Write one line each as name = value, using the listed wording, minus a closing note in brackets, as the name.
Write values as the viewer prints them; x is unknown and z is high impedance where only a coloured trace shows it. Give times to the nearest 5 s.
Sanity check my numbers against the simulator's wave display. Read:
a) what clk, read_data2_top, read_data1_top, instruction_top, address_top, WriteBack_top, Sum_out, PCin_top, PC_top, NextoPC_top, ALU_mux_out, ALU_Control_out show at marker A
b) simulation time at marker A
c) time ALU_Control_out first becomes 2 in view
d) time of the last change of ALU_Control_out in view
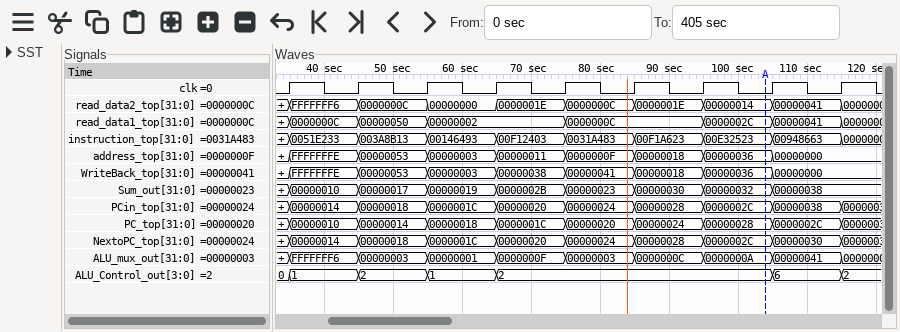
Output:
what clk, read_data2_top, read_data1_top, instruction_top, address_top, WriteBack_top, Sum_out, PCin_top, PC_top, NextoPC_top, ALU_mux_out, ALU_Control_out show at marker A = clk=0, read_data2_top=00000014, read_data1_top=0000002C, instruction_top=00E32523, address_top=00000036, WriteBack_top=00000036, Sum_out=00000032, PCin_top=0000002C, PC_top=00000028, NextoPC_top=0000002C, ALU_mux_out=0000000A, ALU_Control_out=2
simulation time at marker A = 105 s
time ALU_Control_out first becomes 2 in view = 45 s
time of the last change of ALU_Control_out in view = 115 s
